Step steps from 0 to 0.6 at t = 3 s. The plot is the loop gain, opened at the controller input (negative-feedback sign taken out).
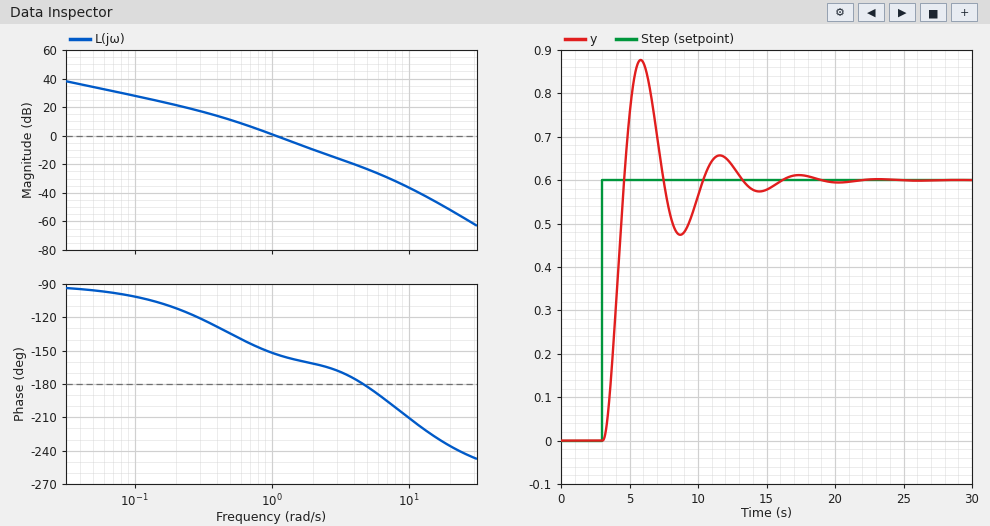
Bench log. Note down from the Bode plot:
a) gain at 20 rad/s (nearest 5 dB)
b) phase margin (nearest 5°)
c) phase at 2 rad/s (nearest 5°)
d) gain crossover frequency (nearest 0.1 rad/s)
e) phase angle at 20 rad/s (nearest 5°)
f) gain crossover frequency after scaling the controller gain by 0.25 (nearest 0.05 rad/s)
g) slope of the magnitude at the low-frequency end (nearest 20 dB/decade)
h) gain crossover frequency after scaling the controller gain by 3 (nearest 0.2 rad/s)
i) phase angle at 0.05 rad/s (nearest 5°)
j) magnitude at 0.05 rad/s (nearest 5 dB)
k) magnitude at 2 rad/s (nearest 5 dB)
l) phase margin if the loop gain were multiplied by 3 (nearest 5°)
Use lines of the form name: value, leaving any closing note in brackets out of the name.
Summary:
gain at 20 rad/s: -50 dB
phase margin: 25°
phase at 2 rad/s: -160°
gain crossover frequency: 1.1 rad/s
phase angle at 20 rad/s: -235°
gain crossover frequency after scaling the controller gain by 0.25: 0.45 rad/s
slope of the magnitude at the low-frequency end: -20 dB/decade
gain crossover frequency after scaling the controller gain by 3: 2.0 rad/s
phase angle at 0.05 rad/s: -95°
magnitude at 0.05 rad/s: 35 dB
magnitude at 2 rad/s: -10 dB
phase margin if the loop gain were multiplied by 3: 20°
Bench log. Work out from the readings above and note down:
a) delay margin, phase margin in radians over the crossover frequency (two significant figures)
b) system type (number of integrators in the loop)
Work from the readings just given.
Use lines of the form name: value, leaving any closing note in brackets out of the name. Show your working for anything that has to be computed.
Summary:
delay margin, phase margin in radians over the crossover frequency: 25 × π / 180 / 1.1 = 0.40 s
system type: 1
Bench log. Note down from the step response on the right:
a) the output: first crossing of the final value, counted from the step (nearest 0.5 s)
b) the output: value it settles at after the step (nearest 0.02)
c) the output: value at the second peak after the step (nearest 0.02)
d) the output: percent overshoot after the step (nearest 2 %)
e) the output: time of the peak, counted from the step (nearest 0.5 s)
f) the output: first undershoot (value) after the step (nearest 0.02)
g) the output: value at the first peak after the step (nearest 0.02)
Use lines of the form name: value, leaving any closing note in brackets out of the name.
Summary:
the output: first crossing of the final value, counted from the step: 1.5 s
the output: value it settles at after the step: 0.60
the output: value at the second peak after the step: 0.66
the output: percent overshoot after the step: 46 %
the output: time of the peak, counted from the step: 3.0 s
the output: first undershoot (value) after the step: 0.48
the output: value at the first peak after the step: 0.88
